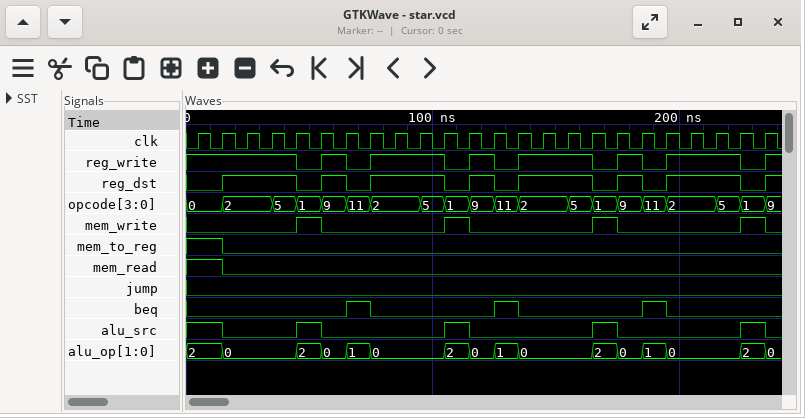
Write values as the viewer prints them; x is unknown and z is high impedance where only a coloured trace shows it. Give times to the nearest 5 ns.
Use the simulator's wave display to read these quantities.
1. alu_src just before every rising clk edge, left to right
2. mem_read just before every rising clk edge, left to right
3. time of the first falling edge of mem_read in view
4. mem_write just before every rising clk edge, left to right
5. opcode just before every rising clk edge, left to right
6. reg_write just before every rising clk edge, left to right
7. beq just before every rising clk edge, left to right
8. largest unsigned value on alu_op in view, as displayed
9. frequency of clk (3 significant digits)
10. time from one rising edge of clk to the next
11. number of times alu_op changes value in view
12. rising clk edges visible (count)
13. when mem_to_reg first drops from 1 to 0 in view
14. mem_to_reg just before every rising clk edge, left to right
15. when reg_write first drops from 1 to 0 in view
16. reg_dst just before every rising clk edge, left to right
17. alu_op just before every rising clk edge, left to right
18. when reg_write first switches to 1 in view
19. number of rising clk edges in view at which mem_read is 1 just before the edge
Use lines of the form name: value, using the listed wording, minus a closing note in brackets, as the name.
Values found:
alu_src just before every rising clk edge, left to right: 1 1 0 0 0 1 0 0 0 0 0 1 0 0 0 0 0 1 0 0 0 0 0 1
mem_read just before every rising clk edge, left to right: 1 1 0 0 0 0 0 0 0 0 0 0 0 0 0 0 0 0 0 0 0 0 0 0
time of the first falling edge of mem_read in view: 15 ns
mem_write just before every rising clk edge, left to right: 0 0 0 0 0 1 0 0 0 0 0 1 0 0 0 0 0 1 0 0 0 0 0 1
opcode just before every rising clk edge, left to right: 0, 0, 2, 2, 5, 1, 9, 11, 2, 2, 5, 1, 9, 11, 2, 2, 5, 1, 9, 11, 2, 2, 5, 1
reg_write just before every rising clk edge, left to right: 1 1 1 1 1 0 1 0 1 1 1 0 1 0 1 1 1 0 1 0 1 1 1 0
beq just before every rising clk edge, left to right: 0 0 0 0 0 0 0 1 0 0 0 0 0 1 0 0 0 0 0 1 0 0 0 0
largest unsigned value on alu_op in view, as displayed: 2
frequency of clk: 100 MHz
time from one rising edge of clk to the next: 10 ns
number of times alu_op changes value in view: 15
rising clk edges visible: 24
when mem_to_reg first drops from 1 to 0 in view: 15 ns
mem_to_reg just before every rising clk edge, left to right: 1 1 0 0 0 0 0 0 0 0 0 0 0 0 0 0 0 0 0 0 0 0 0 0
when reg_write first drops from 1 to 0 in view: 45 ns
reg_dst just before every rising clk edge, left to right: 0 0 1 1 1 0 1 0 1 1 1 0 1 0 1 1 1 0 1 0 1 1 1 0
alu_op just before every rising clk edge, left to right: 2, 2, 0, 0, 0, 2, 0, 1, 0, 0, 0, 2, 0, 1, 0, 0, 0, 2, 0, 1, 0, 0, 0, 2
when reg_write first switches to 1 in view: 55 ns
number of rising clk edges in view at which mem_read is 1 just before the edge: 2
